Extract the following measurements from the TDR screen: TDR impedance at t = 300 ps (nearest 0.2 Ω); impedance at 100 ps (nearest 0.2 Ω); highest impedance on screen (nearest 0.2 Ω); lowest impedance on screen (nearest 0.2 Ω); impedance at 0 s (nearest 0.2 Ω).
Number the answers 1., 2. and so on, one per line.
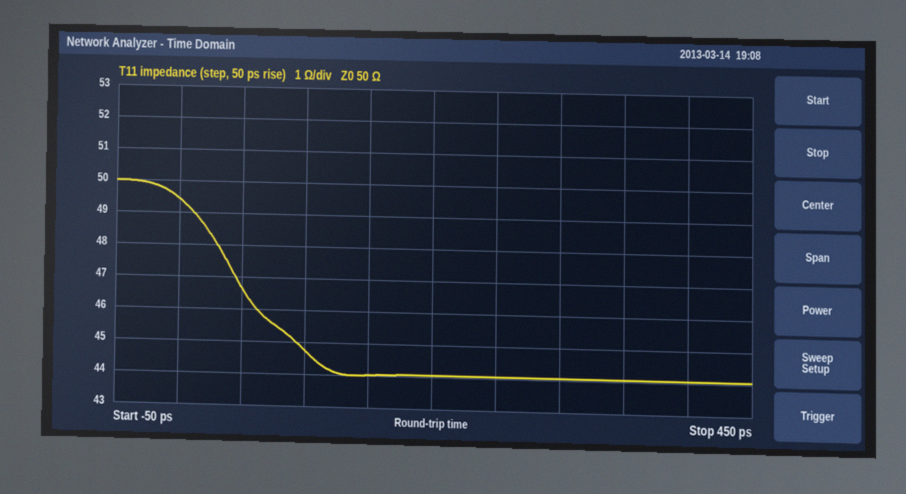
1. 44.0 Ω
2. 44.8 Ω
3. 50.0 Ω
4. 44.0 Ω
5. 49.4 Ω
